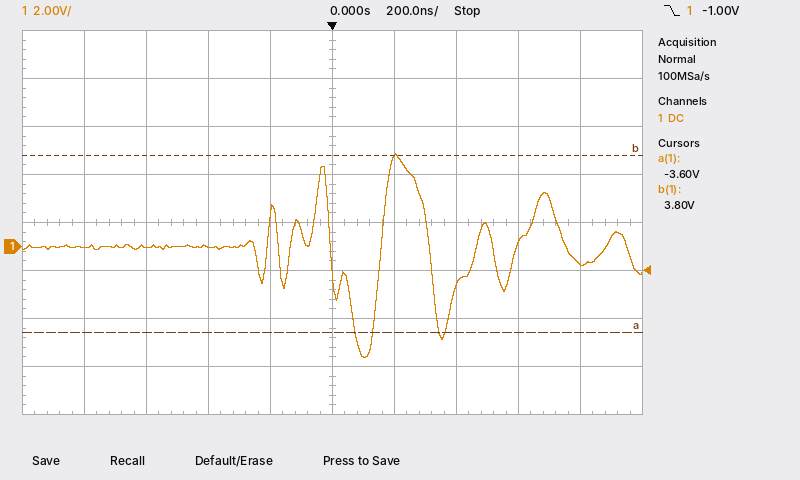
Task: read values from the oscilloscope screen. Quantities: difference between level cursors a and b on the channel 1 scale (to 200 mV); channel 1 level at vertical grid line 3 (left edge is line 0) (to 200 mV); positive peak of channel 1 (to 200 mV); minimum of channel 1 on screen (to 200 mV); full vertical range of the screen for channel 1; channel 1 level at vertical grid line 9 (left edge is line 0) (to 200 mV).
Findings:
7.4 V
0.0 V
3.8 V
-4.6 V
16 V
-800 mV
